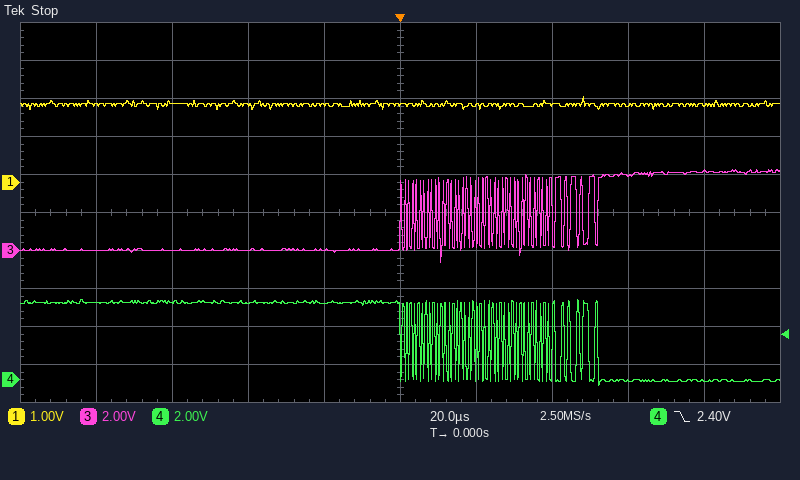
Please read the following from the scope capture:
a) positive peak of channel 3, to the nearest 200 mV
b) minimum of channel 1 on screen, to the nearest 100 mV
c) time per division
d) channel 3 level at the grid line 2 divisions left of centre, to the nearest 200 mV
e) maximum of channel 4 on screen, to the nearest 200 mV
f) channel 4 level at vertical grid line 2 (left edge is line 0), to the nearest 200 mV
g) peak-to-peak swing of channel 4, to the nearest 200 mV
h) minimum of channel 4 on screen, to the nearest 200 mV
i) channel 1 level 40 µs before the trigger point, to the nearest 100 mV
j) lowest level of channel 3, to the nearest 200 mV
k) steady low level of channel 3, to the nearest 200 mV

4.2 V
1.9 V
20 µs
0.0 V
4.2 V
4.0 V
4.6 V
-400 mV
2.0 V
-600 mV
0.0 V
